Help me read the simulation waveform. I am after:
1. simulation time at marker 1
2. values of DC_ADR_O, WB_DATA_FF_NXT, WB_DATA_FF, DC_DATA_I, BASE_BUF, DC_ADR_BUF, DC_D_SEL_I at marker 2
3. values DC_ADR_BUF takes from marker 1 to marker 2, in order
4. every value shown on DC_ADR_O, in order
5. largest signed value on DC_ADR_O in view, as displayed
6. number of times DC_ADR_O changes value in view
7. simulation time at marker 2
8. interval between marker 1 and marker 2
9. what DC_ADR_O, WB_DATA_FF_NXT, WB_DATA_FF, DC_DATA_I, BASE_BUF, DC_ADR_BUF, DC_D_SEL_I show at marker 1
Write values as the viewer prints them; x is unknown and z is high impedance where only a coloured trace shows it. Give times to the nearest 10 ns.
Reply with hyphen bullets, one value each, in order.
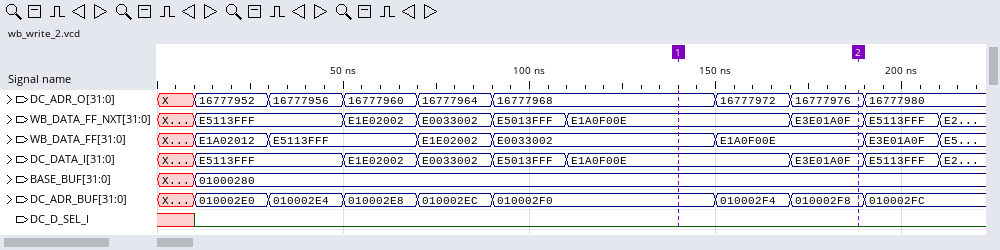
- 140 ns
- DC_ADR_O=16777976, WB_DATA_FF_NXT=E3E01A0F, WB_DATA_FF=E1A0F00E, DC_DATA_I=E3E01A0F, BASE_BUF=01000280, DC_ADR_BUF=010002F8, DC_D_SEL_I=0
- 010002F0, 010002F4, 010002F8
- X, 16777952, 16777956, 16777960, 16777964, 16777968, 16777972, 16777976, 16777980
- 16777980
- 8
- 190 ns
- 50 ns
- DC_ADR_O=16777968, WB_DATA_FF_NXT=E1A0F00E, WB_DATA_FF=E0033002, DC_DATA_I=E1A0F00E, BASE_BUF=01000280, DC_ADR_BUF=010002F0, DC_D_SEL_I=0
